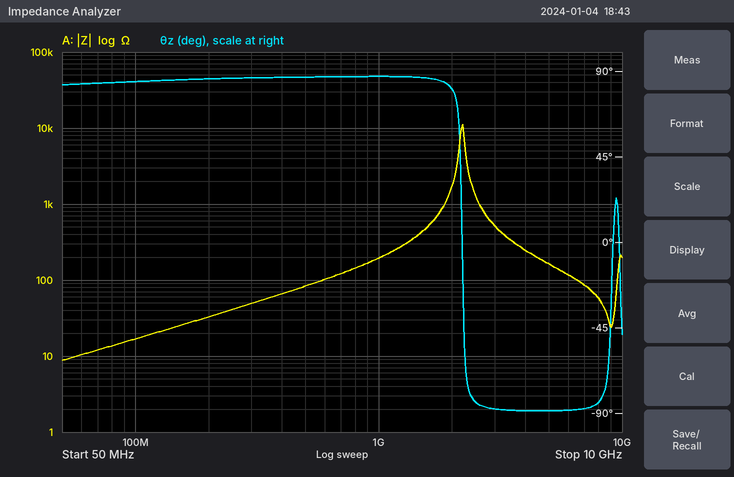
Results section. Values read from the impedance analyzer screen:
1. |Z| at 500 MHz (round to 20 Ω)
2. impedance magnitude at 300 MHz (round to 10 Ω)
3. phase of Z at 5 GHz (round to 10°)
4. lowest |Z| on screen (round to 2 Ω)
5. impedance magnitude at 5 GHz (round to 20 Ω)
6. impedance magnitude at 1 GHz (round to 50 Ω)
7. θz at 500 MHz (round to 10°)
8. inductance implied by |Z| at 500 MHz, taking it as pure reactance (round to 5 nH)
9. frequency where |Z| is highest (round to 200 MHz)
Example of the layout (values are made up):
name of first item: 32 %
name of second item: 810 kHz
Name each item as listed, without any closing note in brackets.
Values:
|Z| at 500 MHz: 80 Ω
impedance magnitude at 300 MHz: 50 Ω
phase of Z at 5 GHz: -90°
lowest |Z| on screen: 8 Ω
impedance magnitude at 5 GHz: 160 Ω
impedance magnitude at 1 GHz: 200 Ω
θz at 500 MHz: 90°
inductance implied by |Z| at 500 MHz, taking it as pure reactance: 25 nH
frequency where |Z| is highest: 2.2 GHz
